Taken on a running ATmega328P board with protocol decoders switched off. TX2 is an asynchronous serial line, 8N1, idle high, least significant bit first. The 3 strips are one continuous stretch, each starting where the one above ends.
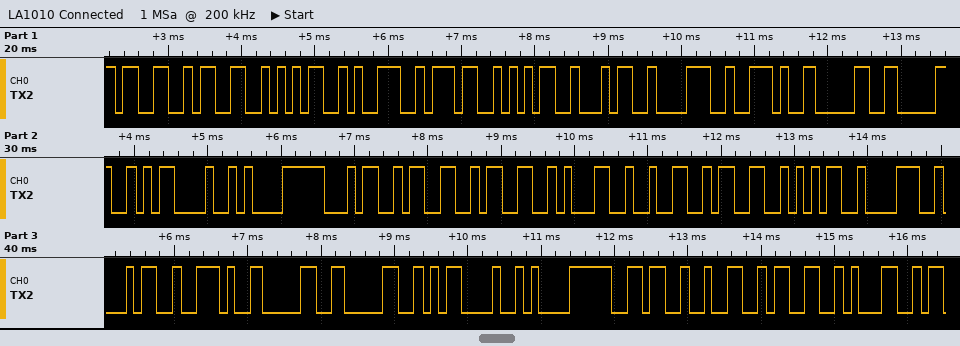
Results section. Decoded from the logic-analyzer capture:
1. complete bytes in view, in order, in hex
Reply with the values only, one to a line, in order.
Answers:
33 33 35 39 37 35 34 38 2E 30 30 0D 0A 34 33 33 31 32 33 35 38 34 2E 30 30 0D 0A 36 32 33 31
